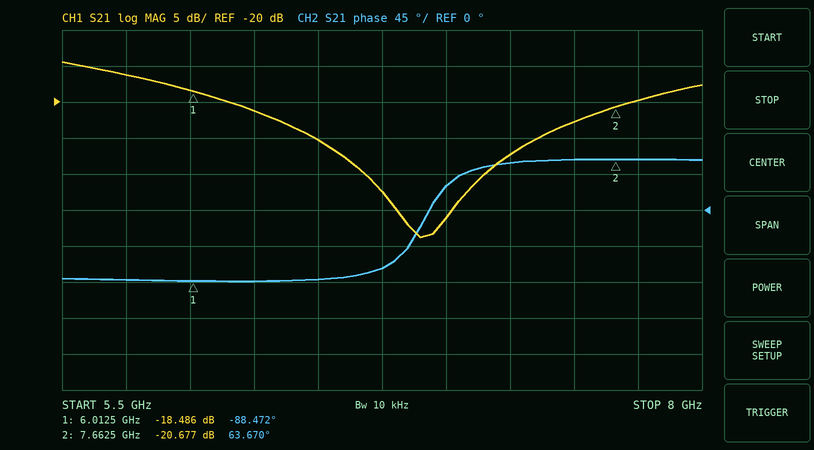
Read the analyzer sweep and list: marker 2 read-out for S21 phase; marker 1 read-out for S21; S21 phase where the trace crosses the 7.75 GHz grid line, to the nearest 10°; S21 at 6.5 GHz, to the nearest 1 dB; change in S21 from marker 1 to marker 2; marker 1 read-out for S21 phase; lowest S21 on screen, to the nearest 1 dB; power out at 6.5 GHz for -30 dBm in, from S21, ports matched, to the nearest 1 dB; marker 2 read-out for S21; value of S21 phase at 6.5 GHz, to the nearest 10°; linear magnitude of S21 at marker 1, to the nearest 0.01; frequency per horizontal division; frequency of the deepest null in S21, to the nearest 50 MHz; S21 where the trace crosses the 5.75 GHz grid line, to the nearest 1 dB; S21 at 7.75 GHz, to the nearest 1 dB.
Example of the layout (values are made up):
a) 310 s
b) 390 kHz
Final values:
a) 63.670°
b) -18.486 dB
c) 60°
d) -25 dB
e) -2.191 dB
f) -88.472°
g) -39 dB
h) -55 dBm
i) -20.677 dB
j) -90°
k) 0.12
l) 250 MHz
m) 6.90 GHz
n) -16 dB
o) -20 dB
